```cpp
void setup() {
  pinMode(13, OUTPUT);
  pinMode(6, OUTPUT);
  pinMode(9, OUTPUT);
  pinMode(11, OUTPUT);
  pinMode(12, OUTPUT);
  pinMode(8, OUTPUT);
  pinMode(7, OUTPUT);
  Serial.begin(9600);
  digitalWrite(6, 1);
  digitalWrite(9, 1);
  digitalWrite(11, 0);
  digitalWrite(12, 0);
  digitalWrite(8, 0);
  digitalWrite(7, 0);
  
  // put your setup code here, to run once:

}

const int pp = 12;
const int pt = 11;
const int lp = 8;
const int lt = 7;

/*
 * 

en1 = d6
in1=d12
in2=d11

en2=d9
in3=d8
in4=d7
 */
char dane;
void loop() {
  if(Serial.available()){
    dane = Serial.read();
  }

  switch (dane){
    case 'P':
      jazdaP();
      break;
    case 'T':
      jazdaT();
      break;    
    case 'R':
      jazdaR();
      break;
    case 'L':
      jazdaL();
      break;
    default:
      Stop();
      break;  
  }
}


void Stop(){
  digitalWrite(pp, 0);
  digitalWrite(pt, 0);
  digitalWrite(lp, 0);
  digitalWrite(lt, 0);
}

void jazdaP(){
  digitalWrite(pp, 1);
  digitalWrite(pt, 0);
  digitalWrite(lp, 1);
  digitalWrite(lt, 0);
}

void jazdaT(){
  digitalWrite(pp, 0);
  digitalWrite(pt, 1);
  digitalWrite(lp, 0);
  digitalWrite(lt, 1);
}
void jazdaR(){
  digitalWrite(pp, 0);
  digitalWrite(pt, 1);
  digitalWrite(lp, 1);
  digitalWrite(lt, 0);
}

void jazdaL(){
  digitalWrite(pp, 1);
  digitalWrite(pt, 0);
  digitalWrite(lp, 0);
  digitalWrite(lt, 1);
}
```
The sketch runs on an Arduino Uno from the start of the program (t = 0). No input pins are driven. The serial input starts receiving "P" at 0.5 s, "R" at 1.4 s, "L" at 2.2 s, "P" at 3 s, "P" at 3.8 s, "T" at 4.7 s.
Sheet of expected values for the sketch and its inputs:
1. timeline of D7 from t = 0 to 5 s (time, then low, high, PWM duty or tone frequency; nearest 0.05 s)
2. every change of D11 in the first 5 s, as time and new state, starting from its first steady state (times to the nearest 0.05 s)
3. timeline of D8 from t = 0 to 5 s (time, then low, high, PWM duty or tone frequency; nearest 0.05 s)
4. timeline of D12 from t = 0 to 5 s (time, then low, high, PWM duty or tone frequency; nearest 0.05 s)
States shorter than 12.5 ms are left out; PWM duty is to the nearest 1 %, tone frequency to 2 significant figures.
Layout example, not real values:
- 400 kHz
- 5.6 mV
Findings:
- 0 s low; 2.2 s high; 3 s low; 4.7 s high
- 0 s low; 1.4 s high; 2.2 s low; 4.7 s high
- 0 s low; 0.5 s high; 2.2 s low; 3 s high; 4.7 s low
- 0 s low; 0.5 s high; 1.4 s low; 2.2 s high; 4.7 s low
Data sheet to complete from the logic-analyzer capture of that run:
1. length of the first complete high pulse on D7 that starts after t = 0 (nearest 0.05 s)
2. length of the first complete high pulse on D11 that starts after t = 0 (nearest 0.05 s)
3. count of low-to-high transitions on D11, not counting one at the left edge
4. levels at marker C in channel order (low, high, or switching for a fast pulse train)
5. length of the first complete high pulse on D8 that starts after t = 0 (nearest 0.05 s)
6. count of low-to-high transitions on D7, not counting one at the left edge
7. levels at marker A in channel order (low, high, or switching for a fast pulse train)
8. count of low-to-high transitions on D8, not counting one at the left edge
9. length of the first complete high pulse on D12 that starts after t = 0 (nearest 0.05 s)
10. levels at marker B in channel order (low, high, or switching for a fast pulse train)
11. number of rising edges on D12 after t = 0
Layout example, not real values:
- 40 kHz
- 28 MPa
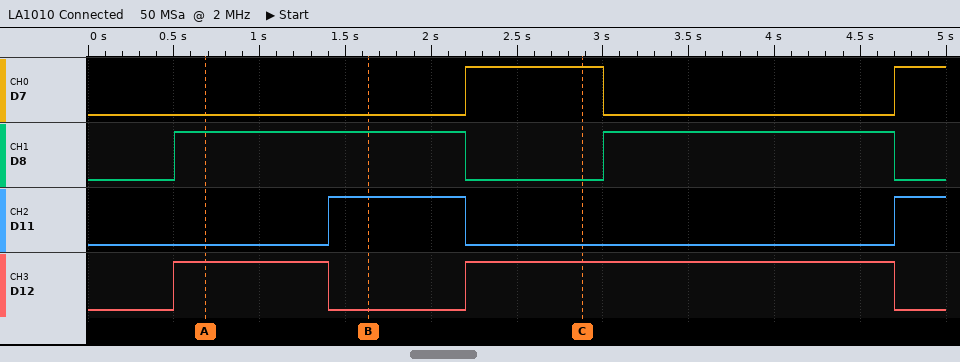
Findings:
- 0.80 s
- 0.80 s
- 2
- D7 high, D8 low, D11 low, D12 high
- 1.70 s
- 2
- D7 low, D8 high, D11 low, D12 high
- 2
- 0.90 s
- D7 low, D8 high, D11 high, D12 low
- 2
